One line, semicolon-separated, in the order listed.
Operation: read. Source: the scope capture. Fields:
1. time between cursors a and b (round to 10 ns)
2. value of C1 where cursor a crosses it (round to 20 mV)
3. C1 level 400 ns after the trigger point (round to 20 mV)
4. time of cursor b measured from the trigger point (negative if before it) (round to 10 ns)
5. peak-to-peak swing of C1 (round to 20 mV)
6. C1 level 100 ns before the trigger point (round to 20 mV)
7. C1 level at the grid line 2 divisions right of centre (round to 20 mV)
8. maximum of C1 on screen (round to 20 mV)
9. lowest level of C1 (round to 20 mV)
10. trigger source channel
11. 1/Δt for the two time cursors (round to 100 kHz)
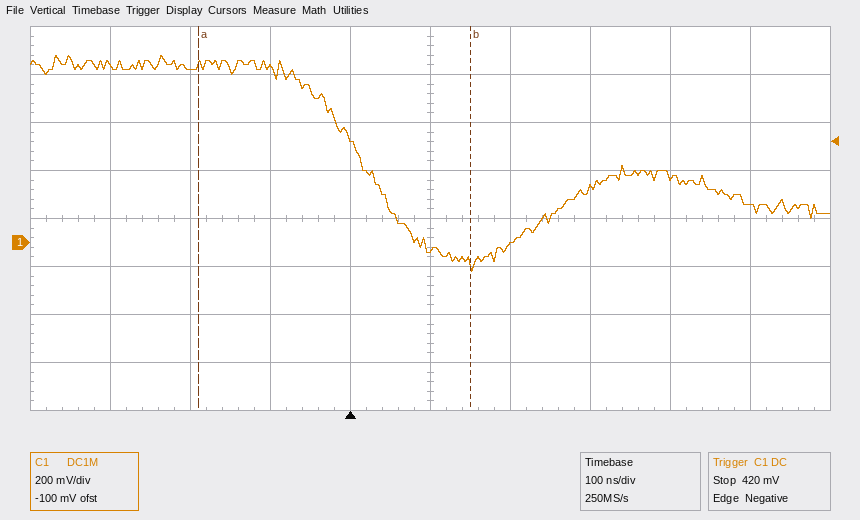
340 ns; 740 mV; 280 mV; +150 ns; 900 mV; 720 mV; 220 mV; 780 mV; -120 mV; C1; 2.9 MHz
